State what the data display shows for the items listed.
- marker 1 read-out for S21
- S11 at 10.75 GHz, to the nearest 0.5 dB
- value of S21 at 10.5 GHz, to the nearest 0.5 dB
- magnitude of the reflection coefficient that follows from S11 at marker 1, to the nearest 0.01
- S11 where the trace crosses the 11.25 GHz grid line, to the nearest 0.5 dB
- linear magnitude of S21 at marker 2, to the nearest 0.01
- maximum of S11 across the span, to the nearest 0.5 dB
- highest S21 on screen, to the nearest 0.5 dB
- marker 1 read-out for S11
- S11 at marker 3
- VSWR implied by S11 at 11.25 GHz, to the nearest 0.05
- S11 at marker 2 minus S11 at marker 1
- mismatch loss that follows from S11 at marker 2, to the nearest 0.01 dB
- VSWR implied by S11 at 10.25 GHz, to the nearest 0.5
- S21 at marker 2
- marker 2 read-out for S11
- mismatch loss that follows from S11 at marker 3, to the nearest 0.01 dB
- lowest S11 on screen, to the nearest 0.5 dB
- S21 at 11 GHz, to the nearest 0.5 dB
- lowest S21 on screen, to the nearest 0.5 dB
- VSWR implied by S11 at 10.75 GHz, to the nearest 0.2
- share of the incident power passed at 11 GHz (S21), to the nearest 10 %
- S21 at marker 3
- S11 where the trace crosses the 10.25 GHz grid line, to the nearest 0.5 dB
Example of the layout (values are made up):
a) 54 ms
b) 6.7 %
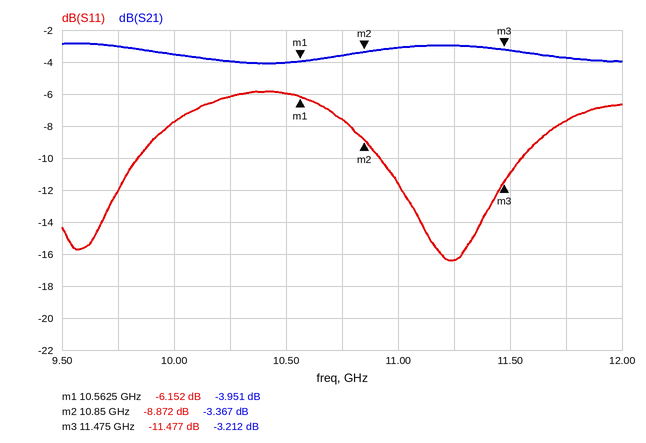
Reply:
a) -3.951 dB
b) -7.5 dB
c) -4.0 dB
d) 0.49
e) -16.5 dB
f) 0.68
g) -6.0 dB
h) -3.0 dB
i) -6.152 dB
j) -11.477 dB
k) 1.35
l) -2.720 dB
m) 0.60 dB
n) 3.0
o) -3.367 dB
p) -8.872 dB
q) 0.32 dB
r) -16.5 dB
s) -3.0 dB
t) -4.0 dB
u) 2.4
v) 50 %
w) -3.212 dB
x) -6.0 dB
